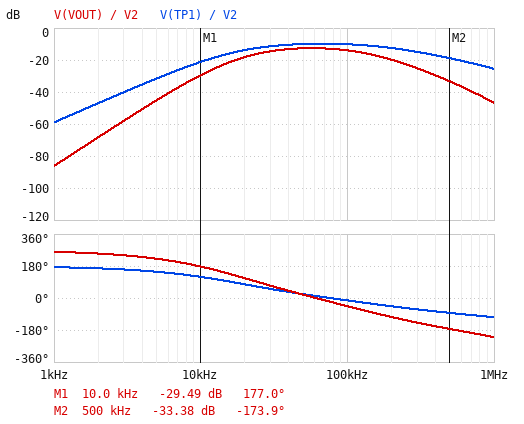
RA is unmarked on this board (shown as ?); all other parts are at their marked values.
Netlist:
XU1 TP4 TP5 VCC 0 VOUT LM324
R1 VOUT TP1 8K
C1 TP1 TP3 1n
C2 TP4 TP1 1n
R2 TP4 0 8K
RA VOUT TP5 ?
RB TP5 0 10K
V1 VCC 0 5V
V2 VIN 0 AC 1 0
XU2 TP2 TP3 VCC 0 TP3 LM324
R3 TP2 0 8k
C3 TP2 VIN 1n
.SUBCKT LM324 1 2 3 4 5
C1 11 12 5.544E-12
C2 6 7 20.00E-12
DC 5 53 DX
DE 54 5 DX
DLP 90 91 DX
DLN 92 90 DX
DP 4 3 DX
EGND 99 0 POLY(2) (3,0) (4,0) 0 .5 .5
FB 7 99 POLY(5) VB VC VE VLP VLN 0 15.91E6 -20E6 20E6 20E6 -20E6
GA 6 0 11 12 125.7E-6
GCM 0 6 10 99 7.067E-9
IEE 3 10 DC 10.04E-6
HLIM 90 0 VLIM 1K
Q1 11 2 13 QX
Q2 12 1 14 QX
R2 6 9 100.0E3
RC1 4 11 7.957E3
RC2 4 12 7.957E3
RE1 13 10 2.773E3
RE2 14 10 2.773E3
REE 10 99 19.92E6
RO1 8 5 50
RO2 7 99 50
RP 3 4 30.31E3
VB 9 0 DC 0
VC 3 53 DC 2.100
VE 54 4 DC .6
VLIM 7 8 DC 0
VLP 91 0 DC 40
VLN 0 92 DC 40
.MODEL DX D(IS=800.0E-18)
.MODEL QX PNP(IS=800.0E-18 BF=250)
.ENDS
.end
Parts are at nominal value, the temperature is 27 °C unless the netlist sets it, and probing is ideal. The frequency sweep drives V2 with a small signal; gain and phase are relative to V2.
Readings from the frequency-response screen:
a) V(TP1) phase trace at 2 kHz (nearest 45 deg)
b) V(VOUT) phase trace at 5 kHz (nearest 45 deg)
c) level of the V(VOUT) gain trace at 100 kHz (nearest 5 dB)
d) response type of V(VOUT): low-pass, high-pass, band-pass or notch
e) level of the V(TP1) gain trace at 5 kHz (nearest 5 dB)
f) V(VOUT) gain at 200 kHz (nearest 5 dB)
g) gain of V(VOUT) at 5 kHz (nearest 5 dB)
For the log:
180 deg
225 deg
-15 dB
band-pass
-30 dB
-20 dB
-45 dB
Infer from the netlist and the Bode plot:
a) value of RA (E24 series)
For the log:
13 kΩ
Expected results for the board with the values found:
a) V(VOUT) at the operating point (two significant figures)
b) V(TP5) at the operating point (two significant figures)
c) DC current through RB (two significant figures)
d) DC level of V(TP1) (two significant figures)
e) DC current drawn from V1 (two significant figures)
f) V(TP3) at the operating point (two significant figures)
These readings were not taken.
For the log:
43 mV
19 mV
1.9 µA
43 mV
350 µA
30 mV
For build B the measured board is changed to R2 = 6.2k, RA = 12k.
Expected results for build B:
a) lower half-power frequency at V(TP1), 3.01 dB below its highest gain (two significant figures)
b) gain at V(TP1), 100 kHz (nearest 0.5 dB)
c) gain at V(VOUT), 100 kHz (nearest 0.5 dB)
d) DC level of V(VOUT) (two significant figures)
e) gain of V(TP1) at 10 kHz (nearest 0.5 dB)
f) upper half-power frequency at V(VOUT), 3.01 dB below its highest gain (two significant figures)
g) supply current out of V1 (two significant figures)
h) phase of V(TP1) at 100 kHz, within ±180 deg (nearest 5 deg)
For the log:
25 kHz
-10.5 dB
-14.5 dB
42 mV
-22.0 dB
140 kHz
350 µA
-10 deg
